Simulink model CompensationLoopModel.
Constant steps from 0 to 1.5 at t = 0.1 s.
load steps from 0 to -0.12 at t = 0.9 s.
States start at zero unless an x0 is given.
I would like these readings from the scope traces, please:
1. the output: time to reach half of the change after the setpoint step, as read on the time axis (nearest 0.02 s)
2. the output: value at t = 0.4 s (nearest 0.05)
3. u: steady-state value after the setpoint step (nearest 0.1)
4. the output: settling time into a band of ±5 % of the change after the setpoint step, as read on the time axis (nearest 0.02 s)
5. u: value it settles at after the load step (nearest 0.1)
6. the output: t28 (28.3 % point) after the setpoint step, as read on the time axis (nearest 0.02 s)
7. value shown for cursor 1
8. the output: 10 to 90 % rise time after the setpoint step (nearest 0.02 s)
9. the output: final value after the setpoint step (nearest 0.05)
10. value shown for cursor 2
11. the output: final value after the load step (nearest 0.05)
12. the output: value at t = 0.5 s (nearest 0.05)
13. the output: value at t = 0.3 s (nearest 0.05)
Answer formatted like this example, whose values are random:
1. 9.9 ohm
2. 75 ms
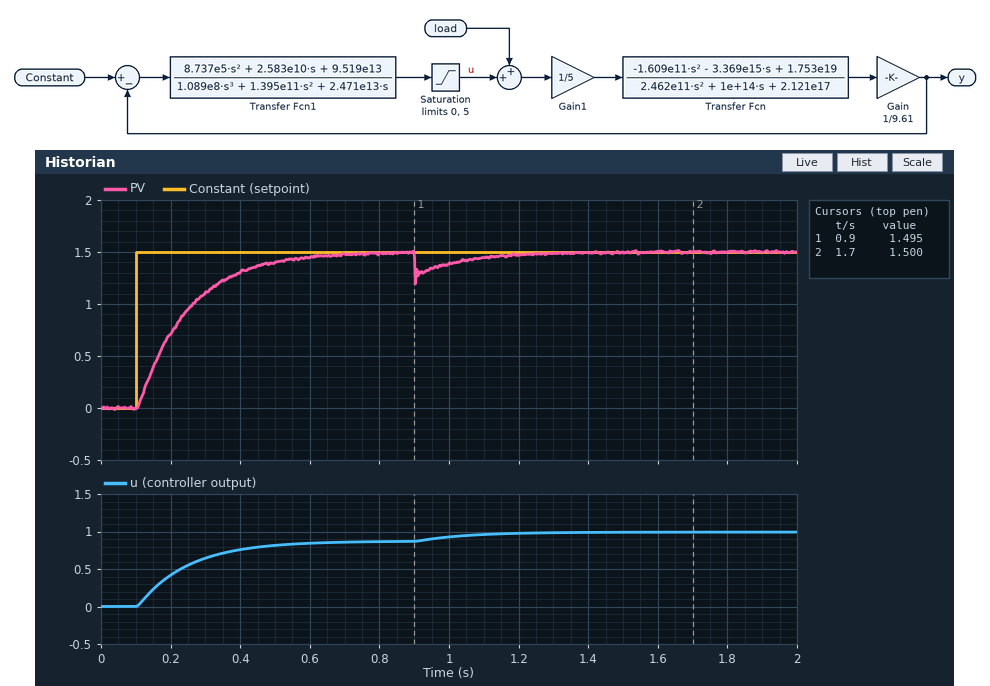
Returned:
1. 0.20 s
2. 1.30
3. 0.9
4. 0.54 s
5. 1.0
6. 0.16 s
7. 1.495
8. 0.32 s
9. 1.50
10. 1.500
11. 1.50
12. 1.40
13. 1.10
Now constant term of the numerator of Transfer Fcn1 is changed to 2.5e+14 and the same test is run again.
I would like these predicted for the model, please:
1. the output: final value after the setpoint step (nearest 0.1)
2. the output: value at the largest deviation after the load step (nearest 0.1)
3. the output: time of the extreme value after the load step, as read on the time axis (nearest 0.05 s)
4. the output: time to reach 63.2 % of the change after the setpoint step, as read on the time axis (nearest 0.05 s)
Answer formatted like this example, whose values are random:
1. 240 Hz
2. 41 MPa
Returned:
1. 1.5
2. 1.2
3. 0.90 s
4. 0.15 s
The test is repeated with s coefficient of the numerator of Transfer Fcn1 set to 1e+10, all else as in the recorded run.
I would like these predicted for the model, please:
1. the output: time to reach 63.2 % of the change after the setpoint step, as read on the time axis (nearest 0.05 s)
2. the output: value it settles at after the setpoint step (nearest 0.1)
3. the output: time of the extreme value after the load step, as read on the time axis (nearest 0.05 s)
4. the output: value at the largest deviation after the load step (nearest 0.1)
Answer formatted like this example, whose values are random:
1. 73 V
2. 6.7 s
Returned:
1. 0.25 s
2. 1.5
3. 0.90 s
4. 1.2
